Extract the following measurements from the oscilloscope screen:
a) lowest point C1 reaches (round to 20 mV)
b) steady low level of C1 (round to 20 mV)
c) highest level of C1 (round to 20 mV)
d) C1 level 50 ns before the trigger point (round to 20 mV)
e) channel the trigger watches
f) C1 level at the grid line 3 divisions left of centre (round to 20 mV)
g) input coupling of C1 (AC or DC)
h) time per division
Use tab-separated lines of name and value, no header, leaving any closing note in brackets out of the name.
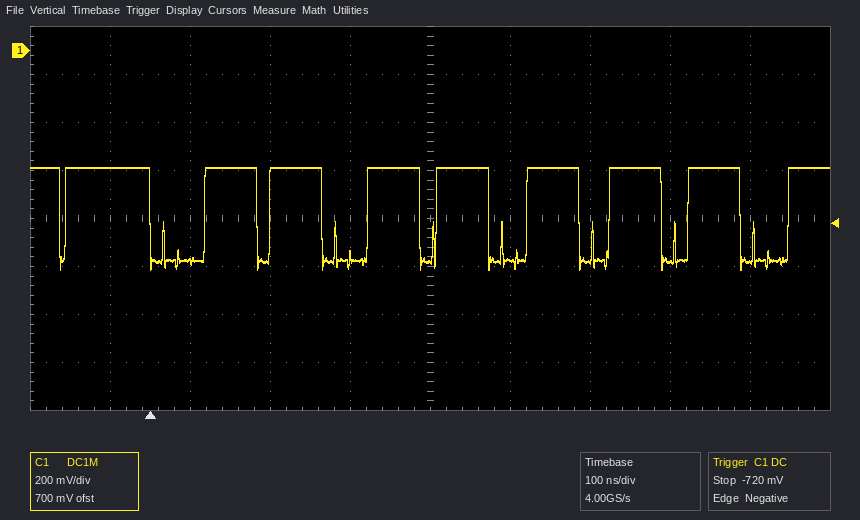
lowest point C1 reaches	-920 mV
steady low level of C1	-880 mV
highest level of C1	-480 mV
C1 level 50 ns before the trigger point	-480 mV
channel the trigger watches	C1
C1 level at the grid line 3 divisions left of centre	-880 mV
input coupling of C1	DC
time per division	100 ns
